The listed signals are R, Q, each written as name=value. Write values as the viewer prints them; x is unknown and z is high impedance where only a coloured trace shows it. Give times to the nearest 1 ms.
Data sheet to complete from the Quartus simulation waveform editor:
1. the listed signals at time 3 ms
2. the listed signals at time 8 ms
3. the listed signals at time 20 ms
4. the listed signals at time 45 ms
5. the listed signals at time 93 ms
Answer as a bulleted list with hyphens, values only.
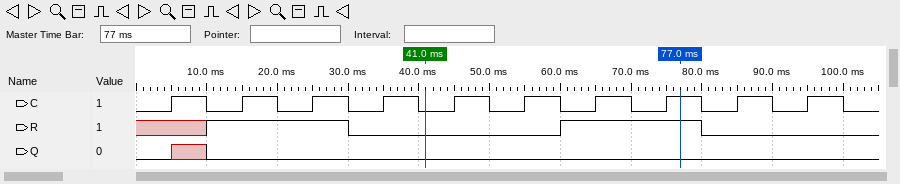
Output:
- R=x, Q=0
- R=x, Q=x
- R=1, Q=0
- R=0, Q=0
- R=0, Q=0
